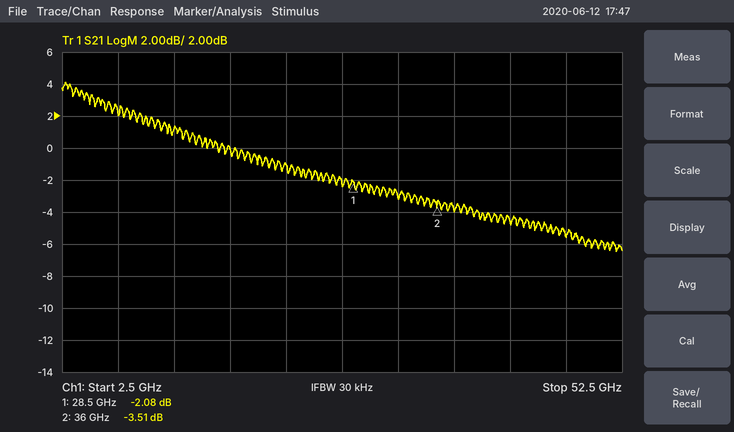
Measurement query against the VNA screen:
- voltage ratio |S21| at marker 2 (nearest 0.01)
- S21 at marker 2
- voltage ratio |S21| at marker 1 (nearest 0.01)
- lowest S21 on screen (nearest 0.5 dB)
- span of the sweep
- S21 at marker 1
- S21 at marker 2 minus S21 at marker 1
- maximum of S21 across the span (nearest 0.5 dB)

0.67
-3.51 dB
0.79
-6.5 dB
50 GHz
-2.08 dB
-1.43 dB
4.0 dB
